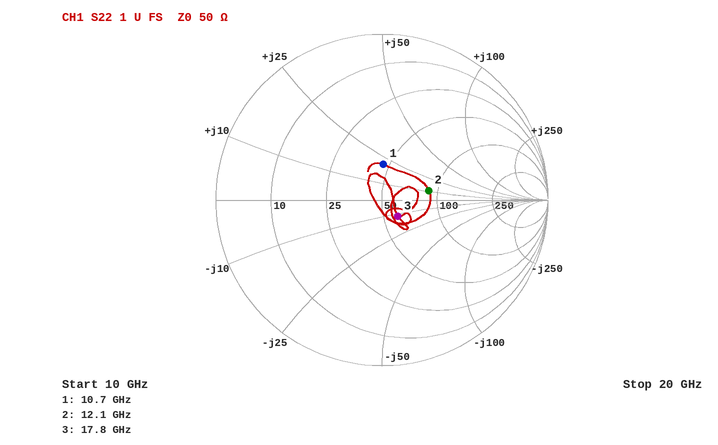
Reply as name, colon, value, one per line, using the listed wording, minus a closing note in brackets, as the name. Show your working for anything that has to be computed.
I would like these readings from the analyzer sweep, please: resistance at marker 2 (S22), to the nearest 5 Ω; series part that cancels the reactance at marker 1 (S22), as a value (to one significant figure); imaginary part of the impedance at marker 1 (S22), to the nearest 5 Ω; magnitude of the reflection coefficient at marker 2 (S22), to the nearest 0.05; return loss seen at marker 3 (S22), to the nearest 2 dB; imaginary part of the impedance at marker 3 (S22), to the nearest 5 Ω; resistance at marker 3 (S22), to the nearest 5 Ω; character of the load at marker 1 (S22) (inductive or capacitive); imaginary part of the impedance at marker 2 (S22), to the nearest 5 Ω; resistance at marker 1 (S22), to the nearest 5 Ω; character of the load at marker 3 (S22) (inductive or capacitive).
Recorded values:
resistance at marker 2 (S22), to the nearest 5 Ω: 90 Ω
series part that cancels the reactance at marker 1 (S22), as a value: C = 1/(2π × 10.7 GHz × 20 Ω) ≈ 744 fF, so 700 fF to one significant figure
imaginary part of the impedance at marker 1 (S22), to the nearest 5 Ω: +20 Ω
magnitude of the reflection coefficient at marker 2 (S22), to the nearest 0.05: 0.30
return loss seen at marker 3 (S22), to the nearest 2 dB: 18 dB
imaginary part of the impedance at marker 3 (S22), to the nearest 5 Ω: -10 Ω
resistance at marker 3 (S22), to the nearest 5 Ω: 60 Ω
character of the load at marker 1 (S22): inductive
imaginary part of the impedance at marker 2 (S22), to the nearest 5 Ω: +10 Ω
resistance at marker 1 (S22), to the nearest 5 Ω: 45 Ω
character of the load at marker 3 (S22): capacitive
